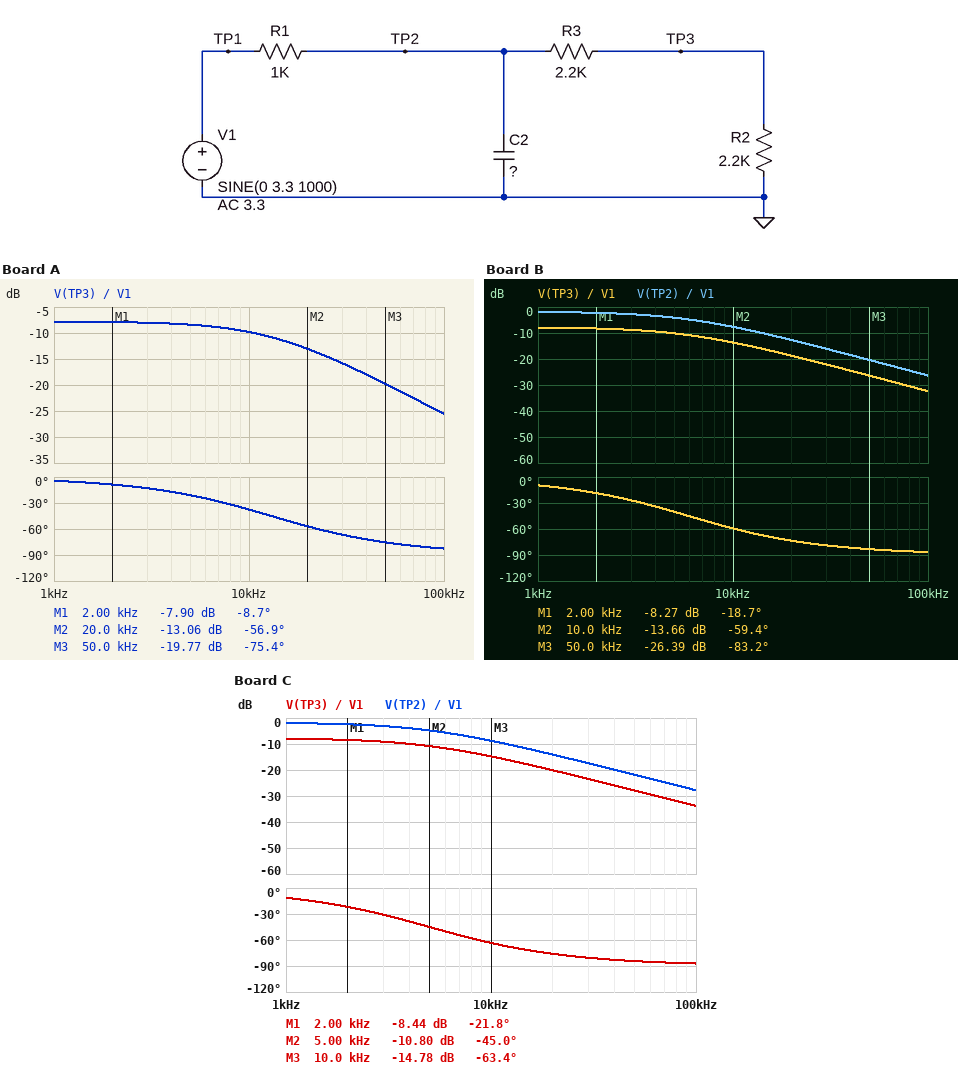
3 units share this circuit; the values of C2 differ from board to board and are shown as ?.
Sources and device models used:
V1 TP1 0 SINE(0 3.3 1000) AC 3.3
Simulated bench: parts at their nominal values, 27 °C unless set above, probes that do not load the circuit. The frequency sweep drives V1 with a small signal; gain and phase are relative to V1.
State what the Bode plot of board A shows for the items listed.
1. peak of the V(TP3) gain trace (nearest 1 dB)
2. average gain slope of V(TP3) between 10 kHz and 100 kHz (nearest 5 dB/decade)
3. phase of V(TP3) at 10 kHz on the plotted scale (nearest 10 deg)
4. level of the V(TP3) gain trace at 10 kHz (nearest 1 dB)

-8 dB
-15 dB/decade
-40 deg
-10 dB
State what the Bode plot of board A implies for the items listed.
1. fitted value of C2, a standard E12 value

15 nF
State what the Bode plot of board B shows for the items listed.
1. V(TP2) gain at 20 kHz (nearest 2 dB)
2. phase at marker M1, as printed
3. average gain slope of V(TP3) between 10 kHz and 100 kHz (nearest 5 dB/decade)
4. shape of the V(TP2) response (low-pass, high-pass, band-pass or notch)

-12 dB
-18.7 deg
-20 dB/decade
low-pass
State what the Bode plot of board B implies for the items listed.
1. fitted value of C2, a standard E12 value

33 nF
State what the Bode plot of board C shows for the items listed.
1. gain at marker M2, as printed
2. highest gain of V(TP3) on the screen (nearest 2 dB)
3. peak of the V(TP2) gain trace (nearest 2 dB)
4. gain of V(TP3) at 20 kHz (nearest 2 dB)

-10.80 dB
-8 dB
-2 dB
-20 dB
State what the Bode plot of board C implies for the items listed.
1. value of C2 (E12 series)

39 nF
